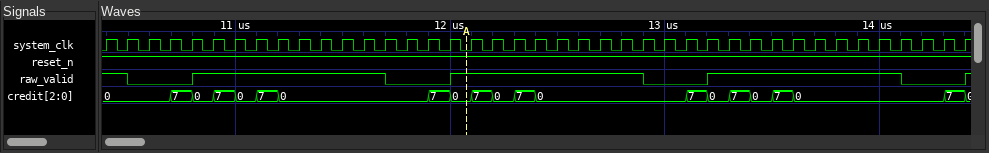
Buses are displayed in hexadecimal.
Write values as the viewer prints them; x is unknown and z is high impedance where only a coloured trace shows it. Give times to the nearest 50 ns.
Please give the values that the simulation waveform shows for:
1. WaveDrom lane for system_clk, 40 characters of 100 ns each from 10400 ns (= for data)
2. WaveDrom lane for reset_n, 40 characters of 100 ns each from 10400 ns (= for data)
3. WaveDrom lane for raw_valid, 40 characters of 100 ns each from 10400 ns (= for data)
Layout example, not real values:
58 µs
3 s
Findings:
{name: 'system_clk', wave: 'p.......................................'}
{name: 'reset_n', wave: '1.......................................'}
{name: 'raw_valid', wave: '10..1........0..1........0..1........0..'}
